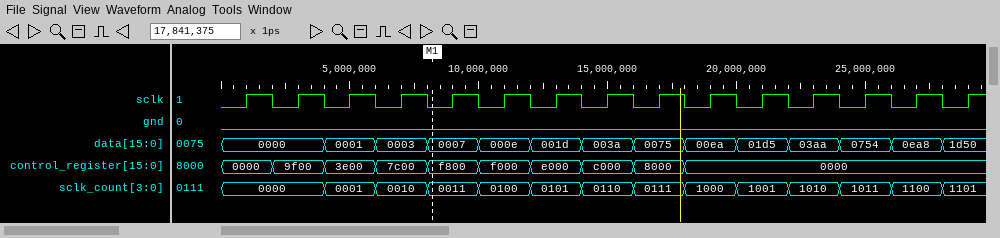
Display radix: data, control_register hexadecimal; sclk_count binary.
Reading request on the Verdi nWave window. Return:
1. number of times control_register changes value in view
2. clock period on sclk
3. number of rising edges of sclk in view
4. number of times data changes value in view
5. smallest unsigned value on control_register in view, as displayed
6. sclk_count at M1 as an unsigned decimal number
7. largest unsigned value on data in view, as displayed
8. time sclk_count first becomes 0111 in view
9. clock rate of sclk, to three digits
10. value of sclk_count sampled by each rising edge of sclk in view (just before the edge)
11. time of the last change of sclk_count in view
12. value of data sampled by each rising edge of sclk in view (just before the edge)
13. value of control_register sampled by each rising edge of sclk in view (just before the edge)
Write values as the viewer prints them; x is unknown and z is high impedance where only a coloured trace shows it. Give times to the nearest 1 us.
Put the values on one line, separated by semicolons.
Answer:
9; 2 us; 15; 13; 0000; 3; 1d50; 16 us; 500 kHz; 0000, 0000, 0001, 0010, 0011, 0100, 0101, 0110, 0111, 1000, 1001, 1010, 1011, 1100, 1101; 28 us; 0000, 0000, 0001, 0003, 0007, 000e, 001d, 003a, 0075, 00ea, 01d5, 03aa, 0754, 0ea8, 1d50; 0000, 9f00, 3e00, 7c00, f800, f000, e000, c000, 8000, 0000, 0000, 0000, 0000, 0000, 0000
